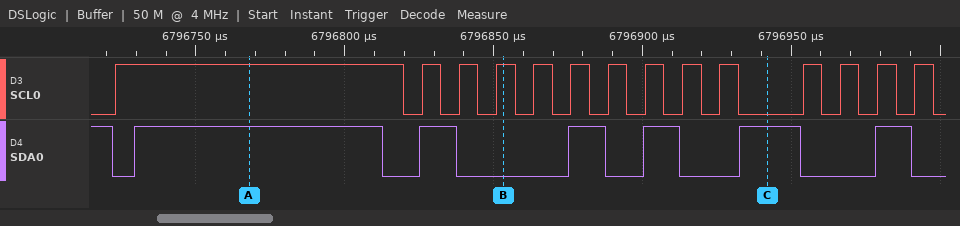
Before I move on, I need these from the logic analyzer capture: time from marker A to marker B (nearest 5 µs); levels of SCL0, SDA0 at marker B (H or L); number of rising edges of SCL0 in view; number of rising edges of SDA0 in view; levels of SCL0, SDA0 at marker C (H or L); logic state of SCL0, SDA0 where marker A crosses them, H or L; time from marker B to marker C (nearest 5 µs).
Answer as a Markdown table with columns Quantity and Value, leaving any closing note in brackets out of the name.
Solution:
| Quantity | Value |
|---|---|
| time from marker A to marker B | 85 µs |
| levels of SCL0, SDA0 at marker B | SCL0=H, SDA0=L |
| number of rising edges of SCL0 in view | 14 |
| number of rising edges of SDA0 in view | 6 |
| levels of SCL0, SDA0 at marker C | SCL0=L, SDA0=H |
| logic state of SCL0, SDA0 where marker A crosses them, H or L | SCL0=H, SDA0=H |
| time from marker B to marker C | 90 µs |
